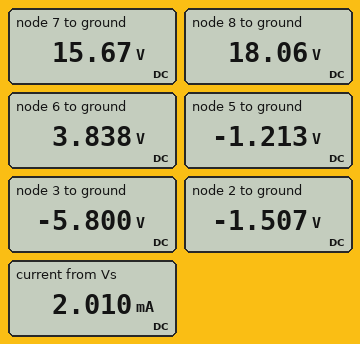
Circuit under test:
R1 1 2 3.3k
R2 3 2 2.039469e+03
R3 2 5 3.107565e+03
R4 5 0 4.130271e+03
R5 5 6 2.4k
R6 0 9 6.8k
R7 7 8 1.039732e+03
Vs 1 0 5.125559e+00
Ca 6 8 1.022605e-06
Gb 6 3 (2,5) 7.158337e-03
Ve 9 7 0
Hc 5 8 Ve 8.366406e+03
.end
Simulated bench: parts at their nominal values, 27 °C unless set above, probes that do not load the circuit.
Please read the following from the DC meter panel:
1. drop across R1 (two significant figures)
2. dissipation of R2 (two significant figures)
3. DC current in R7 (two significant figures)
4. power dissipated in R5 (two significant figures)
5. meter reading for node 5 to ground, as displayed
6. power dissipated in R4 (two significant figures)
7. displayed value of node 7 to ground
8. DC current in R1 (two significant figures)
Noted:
6.6 V
9.0 mW
2.3 mA
11 mW
-1.213 V
360 µW
15.67 V
2.0 mA
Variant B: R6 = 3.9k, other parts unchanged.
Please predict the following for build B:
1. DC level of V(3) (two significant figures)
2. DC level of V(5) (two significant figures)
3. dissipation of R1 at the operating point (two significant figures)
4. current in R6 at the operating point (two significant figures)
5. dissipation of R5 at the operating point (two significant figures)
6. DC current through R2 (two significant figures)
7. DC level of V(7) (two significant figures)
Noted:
6.8 V
6.1 V
300 µW
1.8 mA
240 µW
320 µA
-6.9 V
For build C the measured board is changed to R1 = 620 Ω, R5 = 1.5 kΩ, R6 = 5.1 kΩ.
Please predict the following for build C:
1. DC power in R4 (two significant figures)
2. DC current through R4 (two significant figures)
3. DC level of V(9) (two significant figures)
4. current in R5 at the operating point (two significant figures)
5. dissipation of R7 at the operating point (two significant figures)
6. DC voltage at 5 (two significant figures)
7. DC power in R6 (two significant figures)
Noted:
7.8 mW
1.4 mA
-13 V
1.2 mA
6.8 mW
5.7 V
33 mW
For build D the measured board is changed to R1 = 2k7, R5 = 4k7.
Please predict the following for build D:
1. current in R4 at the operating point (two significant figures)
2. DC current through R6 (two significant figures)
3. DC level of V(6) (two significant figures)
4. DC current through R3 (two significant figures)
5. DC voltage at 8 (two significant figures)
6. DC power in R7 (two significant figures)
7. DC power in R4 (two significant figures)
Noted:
380 µA
3.0 mA
11 V
120 µA
24 V
9.4 mW
610 µW
